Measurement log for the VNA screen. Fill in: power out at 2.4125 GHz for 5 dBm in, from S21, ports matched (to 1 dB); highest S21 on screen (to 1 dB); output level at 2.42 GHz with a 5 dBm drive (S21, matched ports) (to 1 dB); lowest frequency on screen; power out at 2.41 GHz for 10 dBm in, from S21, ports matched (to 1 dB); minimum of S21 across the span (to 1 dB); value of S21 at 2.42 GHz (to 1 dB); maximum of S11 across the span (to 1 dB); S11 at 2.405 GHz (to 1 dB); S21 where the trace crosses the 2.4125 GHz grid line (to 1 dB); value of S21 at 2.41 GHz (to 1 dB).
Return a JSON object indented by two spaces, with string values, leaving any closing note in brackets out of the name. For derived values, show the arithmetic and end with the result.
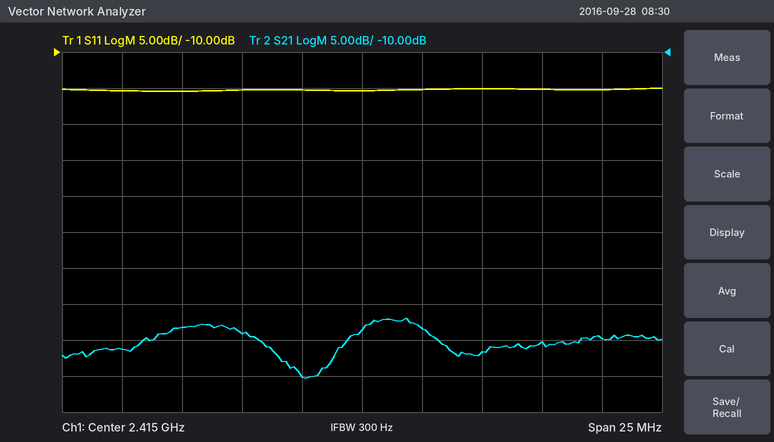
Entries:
{
  "power out at 2.4125 GHz for 5 dBm in, from S21, ports matched": "5 dBm + (-55 dB) = -50 dBm",
  "highest S21 on screen": "-47 dB",
  "output level at 2.42 GHz with a 5 dBm drive (S21, matched ports)": "5 dBm + (-52 dB) = -47 dBm",
  "lowest frequency on screen": "2.4025 GHz",
  "power out at 2.41 GHz for 10 dBm in, from S21, ports matched": "10 dBm + (-49 dB) = -39 dBm",
  "minimum of S21 across the span": "-55 dB",
  "value of S21 at 2.42 GHz": "-52 dB",
  "maximum of S11 across the span": "-15 dB",
  "S11 at 2.405 GHz": "-15 dB",
  "S21 where the trace crosses the 2.4125 GHz grid line": "-55 dB",
  "value of S21 at 2.41 GHz": "-49 dB"
}
